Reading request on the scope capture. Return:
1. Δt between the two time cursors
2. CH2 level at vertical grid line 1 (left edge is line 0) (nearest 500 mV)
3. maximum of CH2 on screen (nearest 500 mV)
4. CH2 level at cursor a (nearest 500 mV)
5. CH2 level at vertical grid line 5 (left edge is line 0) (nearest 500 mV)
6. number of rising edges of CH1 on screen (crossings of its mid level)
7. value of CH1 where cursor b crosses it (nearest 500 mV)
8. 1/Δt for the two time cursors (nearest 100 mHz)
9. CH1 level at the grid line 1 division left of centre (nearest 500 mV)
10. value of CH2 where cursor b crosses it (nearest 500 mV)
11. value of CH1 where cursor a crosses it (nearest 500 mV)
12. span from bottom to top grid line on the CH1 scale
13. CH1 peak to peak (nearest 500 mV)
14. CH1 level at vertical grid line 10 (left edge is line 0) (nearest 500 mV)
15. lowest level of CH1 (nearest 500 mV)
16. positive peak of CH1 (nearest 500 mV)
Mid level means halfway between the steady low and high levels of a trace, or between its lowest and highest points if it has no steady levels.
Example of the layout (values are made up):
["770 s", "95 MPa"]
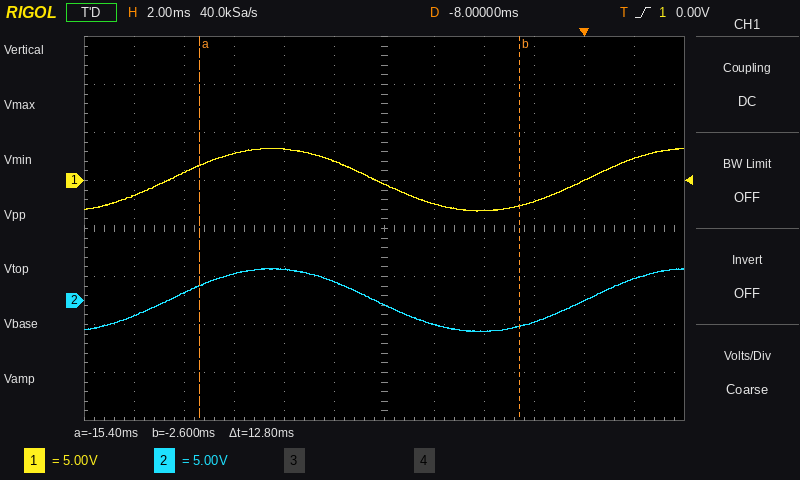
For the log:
["12.8 ms", "-1.5 V", "3.5 V", "1.5 V", "2.0 V", "2", "-2.5 V", "78.1 Hz", "2.0 V", "-2.5 V", "1.5 V", "40 V", "6.5 V", "0.0 V", "-3.0 V", "3.5 V"]
